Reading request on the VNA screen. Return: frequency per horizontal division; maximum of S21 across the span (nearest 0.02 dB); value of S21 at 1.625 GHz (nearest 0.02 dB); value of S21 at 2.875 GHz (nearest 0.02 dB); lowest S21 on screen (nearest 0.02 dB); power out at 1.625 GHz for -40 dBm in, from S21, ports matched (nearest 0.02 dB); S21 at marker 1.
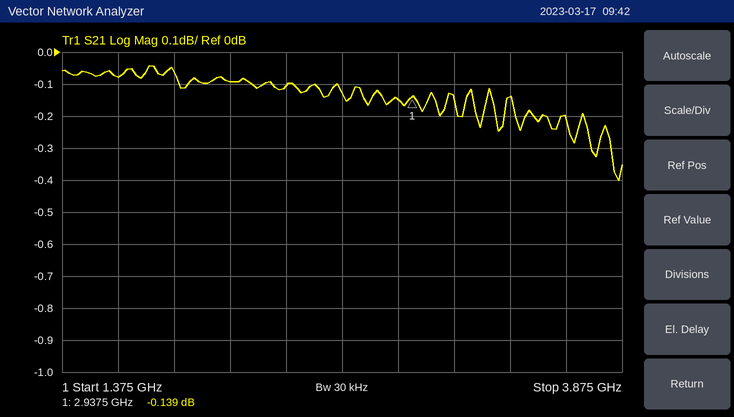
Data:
250 MHz
-0.04 dB
-0.08 dB
-0.14 dB
-0.40 dB
-40.08 dBm
-0.139 dB
